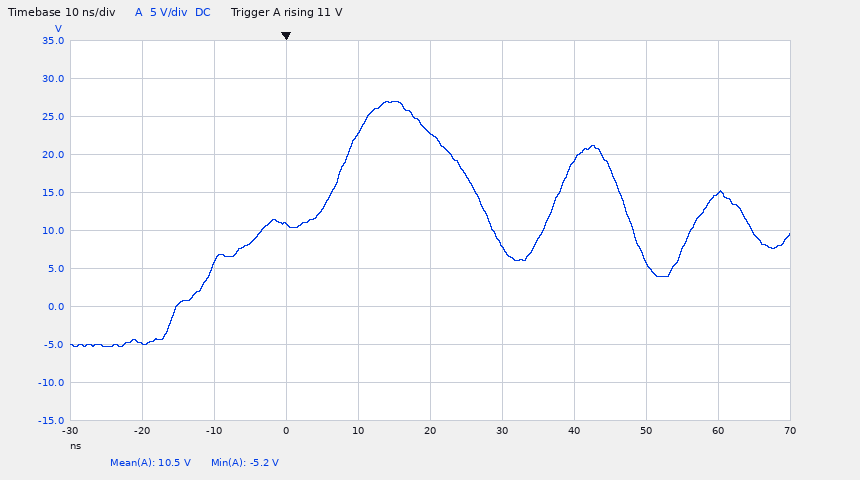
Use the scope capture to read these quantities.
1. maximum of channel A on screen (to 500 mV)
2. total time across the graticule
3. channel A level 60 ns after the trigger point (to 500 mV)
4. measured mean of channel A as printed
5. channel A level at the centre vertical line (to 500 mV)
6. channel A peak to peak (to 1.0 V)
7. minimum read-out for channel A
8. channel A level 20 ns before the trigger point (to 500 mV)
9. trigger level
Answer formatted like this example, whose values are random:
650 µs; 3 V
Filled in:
27.0 V; 100 ns; 15.0 V; 10.5 V; 23.0 V; 32.0 V; -5.2 V; -5.0 V; 11 V
